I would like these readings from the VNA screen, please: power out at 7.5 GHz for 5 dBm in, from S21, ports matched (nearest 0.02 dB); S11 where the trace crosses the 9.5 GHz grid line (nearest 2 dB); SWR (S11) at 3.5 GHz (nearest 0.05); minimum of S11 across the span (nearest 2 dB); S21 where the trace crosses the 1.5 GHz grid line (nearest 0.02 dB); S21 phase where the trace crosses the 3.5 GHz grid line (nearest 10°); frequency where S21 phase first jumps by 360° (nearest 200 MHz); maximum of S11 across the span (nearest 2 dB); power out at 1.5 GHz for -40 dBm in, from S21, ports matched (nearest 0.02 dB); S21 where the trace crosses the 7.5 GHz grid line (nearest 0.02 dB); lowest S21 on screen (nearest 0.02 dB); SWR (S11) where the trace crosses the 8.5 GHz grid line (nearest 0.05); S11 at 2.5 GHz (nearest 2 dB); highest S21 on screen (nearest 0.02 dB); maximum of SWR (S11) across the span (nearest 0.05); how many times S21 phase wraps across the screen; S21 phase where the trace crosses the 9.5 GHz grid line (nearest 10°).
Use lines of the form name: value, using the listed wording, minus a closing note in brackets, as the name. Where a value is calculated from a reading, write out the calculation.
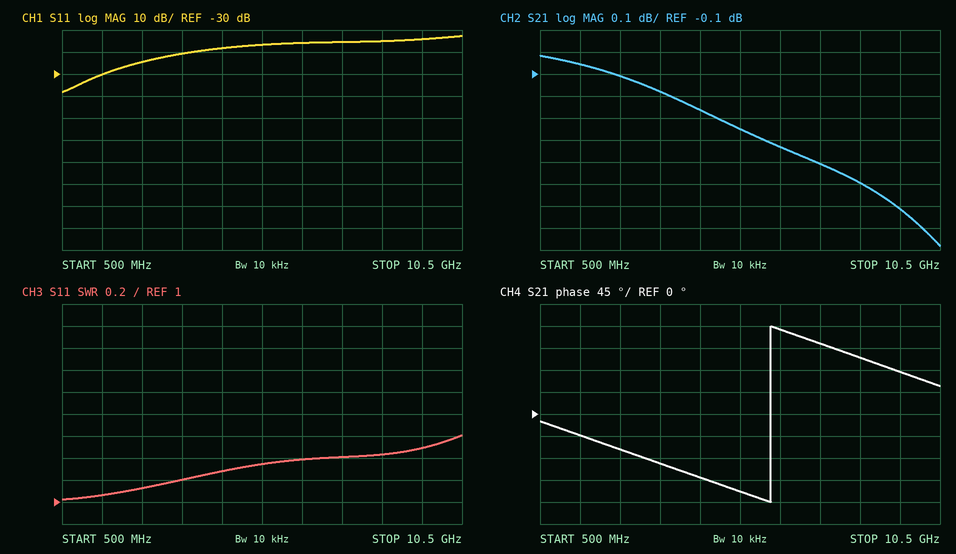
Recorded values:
power out at 7.5 GHz for 5 dBm in, from S21, ports matched: 5 dBm + (-0.50 dB) = 4.50 dBm
S11 where the trace crosses the 9.5 GHz grid line: -14 dB
SWR (S11) at 3.5 GHz: 1.20
minimum of S11 across the span: -38 dB
S21 where the trace crosses the 1.5 GHz grid line: -0.06 dB
S21 phase where the trace crosses the 3.5 GHz grid line: -100°
frequency where S21 phase first jumps by 360°: 6.2 GHz
maximum of S11 across the span: -12 dB
power out at 1.5 GHz for -40 dBm in, from S21, ports matched: -40 dBm + (-0.06 dB) = -40.06 dBm
S21 where the trace crosses the 7.5 GHz grid line: -0.50 dB
lowest S21 on screen: -0.88 dB
SWR (S11) where the trace crosses the 8.5 GHz grid line: 1.45
S11 at 2.5 GHz: -24 dB
highest S21 on screen: -0.02 dB
maximum of SWR (S11) across the span: 1.60
how many times S21 phase wraps across the screen: 1
S21 phase where the trace crosses the 9.5 GHz grid line: 90°
